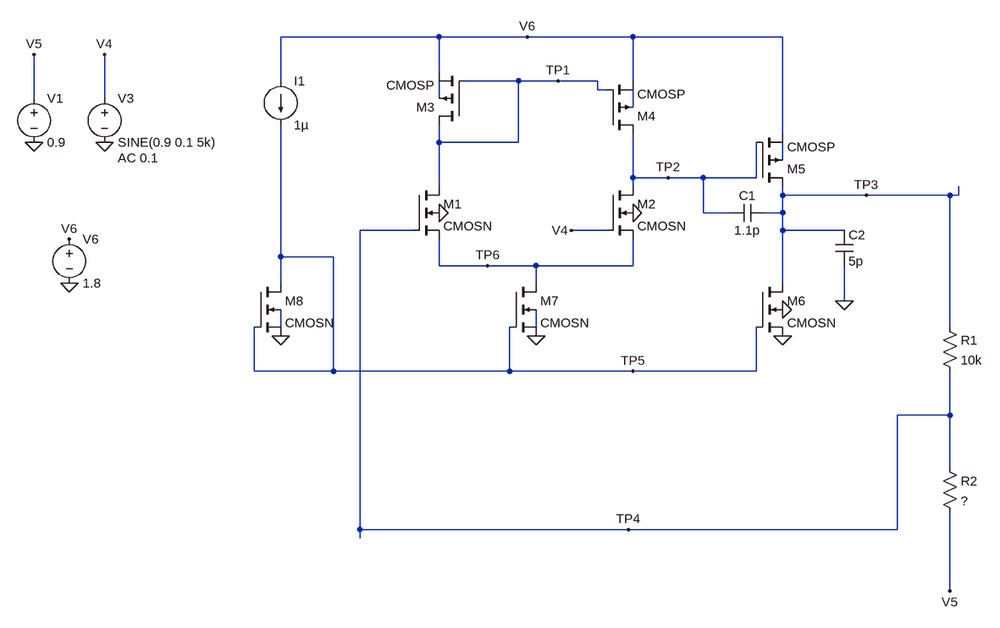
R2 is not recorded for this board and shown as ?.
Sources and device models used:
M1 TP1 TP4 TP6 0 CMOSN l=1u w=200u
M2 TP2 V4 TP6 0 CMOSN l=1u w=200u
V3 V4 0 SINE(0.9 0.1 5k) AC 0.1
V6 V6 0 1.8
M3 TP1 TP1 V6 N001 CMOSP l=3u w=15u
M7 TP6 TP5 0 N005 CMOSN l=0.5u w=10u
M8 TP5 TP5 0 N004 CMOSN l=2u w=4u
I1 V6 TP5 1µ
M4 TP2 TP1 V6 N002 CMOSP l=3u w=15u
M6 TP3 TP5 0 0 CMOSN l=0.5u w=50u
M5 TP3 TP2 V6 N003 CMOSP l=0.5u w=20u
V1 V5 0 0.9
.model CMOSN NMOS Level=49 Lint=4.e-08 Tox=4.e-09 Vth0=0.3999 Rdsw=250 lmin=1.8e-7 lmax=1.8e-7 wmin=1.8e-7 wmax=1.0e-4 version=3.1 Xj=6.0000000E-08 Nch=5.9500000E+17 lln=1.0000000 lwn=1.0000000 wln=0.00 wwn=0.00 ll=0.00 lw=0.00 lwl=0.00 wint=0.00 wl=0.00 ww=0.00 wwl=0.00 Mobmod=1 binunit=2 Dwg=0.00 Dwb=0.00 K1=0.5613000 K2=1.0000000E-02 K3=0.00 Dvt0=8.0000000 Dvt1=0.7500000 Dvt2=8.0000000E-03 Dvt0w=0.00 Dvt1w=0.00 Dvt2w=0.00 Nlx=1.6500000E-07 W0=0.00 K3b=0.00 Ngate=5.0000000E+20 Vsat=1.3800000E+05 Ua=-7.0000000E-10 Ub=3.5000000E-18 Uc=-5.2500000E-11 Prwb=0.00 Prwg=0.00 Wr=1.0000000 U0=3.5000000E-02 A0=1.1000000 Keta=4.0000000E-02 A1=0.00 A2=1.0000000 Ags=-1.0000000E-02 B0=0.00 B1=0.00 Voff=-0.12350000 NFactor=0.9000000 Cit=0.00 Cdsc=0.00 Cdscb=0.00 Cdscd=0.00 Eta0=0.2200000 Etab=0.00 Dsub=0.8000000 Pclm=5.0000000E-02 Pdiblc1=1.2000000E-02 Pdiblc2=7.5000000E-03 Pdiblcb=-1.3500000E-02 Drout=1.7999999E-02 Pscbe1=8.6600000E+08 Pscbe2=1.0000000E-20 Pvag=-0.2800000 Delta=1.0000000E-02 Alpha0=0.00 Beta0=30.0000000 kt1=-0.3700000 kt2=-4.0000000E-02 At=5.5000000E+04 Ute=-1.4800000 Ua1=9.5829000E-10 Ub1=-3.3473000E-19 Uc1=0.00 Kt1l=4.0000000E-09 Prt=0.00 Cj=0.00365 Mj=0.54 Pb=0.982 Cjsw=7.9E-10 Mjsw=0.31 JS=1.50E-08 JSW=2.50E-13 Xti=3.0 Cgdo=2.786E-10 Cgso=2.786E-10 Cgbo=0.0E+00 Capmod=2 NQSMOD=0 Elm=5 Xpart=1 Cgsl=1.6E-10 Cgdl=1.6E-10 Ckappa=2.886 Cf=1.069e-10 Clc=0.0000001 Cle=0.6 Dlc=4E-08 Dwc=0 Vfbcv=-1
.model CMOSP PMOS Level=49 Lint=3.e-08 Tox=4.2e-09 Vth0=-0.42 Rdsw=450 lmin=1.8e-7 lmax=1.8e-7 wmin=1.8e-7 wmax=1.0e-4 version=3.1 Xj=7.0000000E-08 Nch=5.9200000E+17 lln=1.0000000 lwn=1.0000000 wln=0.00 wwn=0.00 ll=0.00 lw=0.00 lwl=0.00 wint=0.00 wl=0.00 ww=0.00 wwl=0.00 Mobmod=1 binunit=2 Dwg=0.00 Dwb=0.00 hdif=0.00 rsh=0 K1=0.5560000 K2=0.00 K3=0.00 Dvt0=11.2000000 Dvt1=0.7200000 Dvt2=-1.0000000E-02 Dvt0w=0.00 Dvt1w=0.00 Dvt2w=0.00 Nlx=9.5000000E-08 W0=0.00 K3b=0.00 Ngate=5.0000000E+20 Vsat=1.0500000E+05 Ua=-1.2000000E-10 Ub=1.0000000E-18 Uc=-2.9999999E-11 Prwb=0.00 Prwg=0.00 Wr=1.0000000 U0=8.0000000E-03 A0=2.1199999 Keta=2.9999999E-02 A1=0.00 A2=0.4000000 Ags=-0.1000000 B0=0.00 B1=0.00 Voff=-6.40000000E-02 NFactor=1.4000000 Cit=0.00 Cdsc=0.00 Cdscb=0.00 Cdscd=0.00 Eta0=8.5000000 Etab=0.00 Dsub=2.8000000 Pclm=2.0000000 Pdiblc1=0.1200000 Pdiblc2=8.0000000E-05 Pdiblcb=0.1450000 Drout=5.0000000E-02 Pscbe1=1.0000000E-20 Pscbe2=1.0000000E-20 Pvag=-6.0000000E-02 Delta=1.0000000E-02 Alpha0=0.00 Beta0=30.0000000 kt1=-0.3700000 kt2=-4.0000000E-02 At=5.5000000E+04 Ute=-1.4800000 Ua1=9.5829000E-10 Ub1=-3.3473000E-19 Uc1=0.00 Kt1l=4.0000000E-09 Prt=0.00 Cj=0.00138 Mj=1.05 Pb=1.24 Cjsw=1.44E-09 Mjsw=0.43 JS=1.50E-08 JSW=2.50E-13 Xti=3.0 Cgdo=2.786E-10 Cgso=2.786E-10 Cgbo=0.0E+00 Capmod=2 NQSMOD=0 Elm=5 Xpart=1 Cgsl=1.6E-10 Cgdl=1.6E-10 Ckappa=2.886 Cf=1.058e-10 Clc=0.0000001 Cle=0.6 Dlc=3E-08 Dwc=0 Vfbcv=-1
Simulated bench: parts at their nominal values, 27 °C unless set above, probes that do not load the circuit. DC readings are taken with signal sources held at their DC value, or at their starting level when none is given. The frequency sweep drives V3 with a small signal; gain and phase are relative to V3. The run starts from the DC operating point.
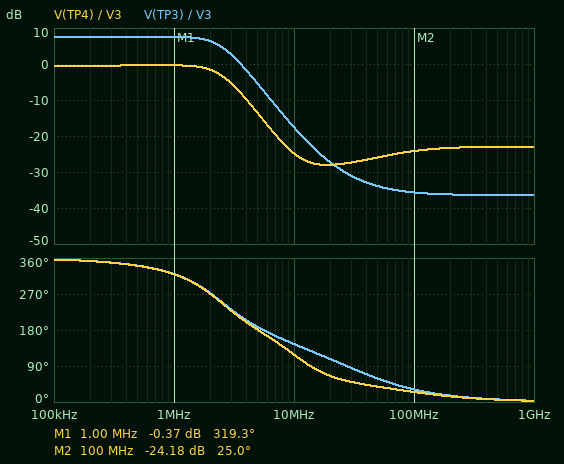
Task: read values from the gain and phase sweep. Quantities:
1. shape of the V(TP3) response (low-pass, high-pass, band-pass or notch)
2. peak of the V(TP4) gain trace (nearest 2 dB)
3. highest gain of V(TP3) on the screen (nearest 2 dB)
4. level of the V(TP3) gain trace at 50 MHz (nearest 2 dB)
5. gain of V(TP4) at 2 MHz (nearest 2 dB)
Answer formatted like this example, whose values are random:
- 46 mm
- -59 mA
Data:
- low-pass
- 0 dB
- 8 dB
- -34 dB
- -2 dB
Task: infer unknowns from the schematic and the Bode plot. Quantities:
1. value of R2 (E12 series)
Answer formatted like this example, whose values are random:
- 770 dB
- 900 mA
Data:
- 6.8 kΩ
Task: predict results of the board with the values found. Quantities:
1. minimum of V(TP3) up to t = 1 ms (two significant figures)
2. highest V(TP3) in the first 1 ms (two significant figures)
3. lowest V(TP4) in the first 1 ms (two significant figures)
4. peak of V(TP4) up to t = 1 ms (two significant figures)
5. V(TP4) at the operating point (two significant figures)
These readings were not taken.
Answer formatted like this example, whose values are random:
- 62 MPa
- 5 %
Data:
- 810 mV
- 1.1 V
- 860 mV
- 1.0 V
- 900 mV
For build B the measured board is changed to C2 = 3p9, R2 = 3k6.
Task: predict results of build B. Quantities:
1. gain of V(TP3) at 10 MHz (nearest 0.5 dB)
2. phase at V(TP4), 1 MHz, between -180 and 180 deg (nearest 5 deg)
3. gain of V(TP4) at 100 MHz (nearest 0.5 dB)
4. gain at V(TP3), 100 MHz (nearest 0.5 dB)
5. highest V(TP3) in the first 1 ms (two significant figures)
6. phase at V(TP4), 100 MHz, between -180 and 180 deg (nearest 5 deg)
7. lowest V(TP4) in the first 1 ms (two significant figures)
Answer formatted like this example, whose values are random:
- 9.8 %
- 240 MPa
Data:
- -16.0 dB
- -55 deg
- -26.0 dB
- -33.5 dB
- 1.3 V
- 35 deg
- 880 mV
